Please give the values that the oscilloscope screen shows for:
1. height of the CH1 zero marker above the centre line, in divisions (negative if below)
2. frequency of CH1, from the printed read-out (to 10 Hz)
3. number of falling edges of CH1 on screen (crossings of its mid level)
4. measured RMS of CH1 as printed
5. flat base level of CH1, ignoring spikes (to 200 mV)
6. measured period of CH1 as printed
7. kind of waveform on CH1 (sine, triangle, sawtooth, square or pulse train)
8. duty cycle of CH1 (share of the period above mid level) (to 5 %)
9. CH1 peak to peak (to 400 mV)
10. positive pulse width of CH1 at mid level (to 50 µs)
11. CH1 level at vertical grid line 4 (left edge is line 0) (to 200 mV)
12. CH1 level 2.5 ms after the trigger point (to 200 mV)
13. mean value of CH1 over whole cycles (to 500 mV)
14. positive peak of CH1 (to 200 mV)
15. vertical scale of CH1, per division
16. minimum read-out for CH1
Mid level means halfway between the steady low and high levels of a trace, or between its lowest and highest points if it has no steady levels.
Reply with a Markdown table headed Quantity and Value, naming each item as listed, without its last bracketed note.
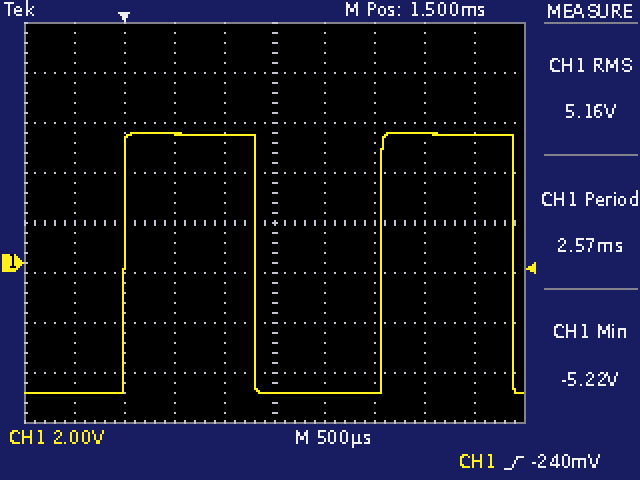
| Quantity | Value |
|---|---|
| height of the CH1 zero marker above the centre line, in divisions | -0.8 div |
| frequency of CH1, from the printed read-out | 390 Hz |
| number of falling edges of CH1 on screen | 2 |
| measured RMS of CH1 as printed | 5.16 V |
| flat base level of CH1, ignoring spikes | -5.2 V |
| measured period of CH1 as printed | 2.57 ms |
| kind of waveform on CH1 | square |
| duty cycle of CH1 (share of the period above mid level) | 50 % |
| CH1 peak to peak | 10.4 V |
| positive pulse width of CH1 at mid level | 1.30 ms |
| CH1 level at vertical grid line 4 (left edge is line 0) | 5.2 V |
| CH1 level 2.5 ms after the trigger point | -5.2 V |
| mean value of CH1 over whole cycles | 0.0 V |
| positive peak of CH1 | 5.2 V |
| vertical scale of CH1, per division | 2 V |
| minimum read-out for CH1 | -5.22 V |
